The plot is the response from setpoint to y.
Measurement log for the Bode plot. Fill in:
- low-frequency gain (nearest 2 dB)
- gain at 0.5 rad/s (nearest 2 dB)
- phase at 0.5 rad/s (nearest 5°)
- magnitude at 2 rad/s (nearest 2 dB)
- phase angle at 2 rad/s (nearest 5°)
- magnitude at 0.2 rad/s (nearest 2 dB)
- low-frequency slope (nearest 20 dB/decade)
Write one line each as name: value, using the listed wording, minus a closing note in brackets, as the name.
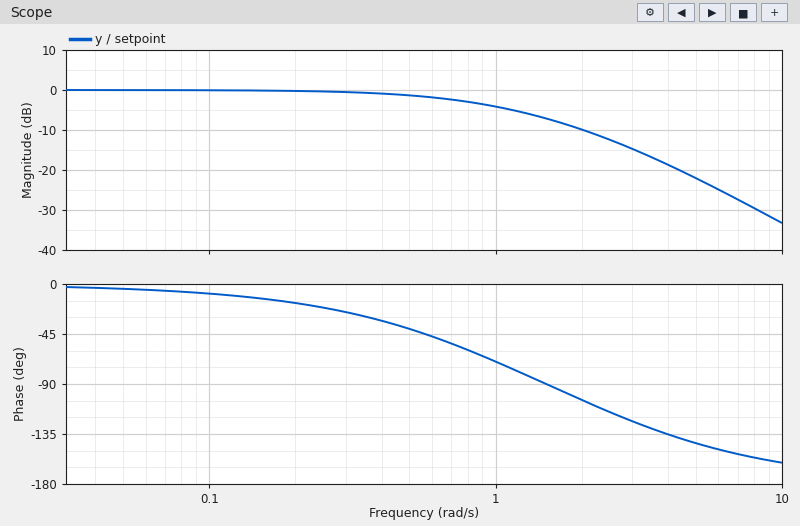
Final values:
low-frequency gain: 0 dB
gain at 0.5 rad/s: -2 dB
phase at 0.5 rad/s: -40°
magnitude at 2 rad/s: -10 dB
phase angle at 2 rad/s: -105°
magnitude at 0.2 rad/s: 0 dB
low-frequency slope: 0 dB/decade
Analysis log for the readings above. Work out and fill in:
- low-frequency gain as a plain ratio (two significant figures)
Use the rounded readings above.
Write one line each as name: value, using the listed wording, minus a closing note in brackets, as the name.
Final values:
low-frequency gain as a plain ratio: 1.0
